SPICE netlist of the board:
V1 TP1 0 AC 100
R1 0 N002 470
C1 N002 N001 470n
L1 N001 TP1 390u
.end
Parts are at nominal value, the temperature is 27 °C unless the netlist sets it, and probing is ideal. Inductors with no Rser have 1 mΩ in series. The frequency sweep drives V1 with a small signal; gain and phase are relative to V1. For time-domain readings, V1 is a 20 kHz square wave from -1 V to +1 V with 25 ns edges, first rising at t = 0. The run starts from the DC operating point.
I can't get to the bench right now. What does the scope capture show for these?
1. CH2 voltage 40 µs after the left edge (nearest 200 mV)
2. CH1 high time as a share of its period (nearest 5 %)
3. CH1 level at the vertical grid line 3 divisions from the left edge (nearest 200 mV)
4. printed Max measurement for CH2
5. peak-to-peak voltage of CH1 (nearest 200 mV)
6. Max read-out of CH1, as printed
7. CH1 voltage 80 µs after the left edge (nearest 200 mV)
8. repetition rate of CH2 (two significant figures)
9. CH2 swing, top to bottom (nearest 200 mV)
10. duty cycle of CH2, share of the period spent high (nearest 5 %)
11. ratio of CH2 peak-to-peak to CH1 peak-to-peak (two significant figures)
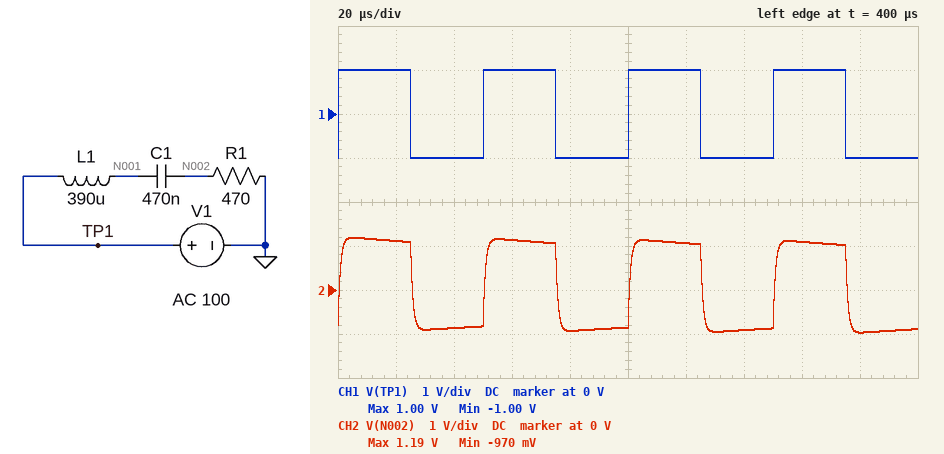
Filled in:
-800 mV
50 %
1.0 V
1.19 V
2.0 V
1.00 V
-1.0 V
20 kHz
2.2 V
50 %
1.1
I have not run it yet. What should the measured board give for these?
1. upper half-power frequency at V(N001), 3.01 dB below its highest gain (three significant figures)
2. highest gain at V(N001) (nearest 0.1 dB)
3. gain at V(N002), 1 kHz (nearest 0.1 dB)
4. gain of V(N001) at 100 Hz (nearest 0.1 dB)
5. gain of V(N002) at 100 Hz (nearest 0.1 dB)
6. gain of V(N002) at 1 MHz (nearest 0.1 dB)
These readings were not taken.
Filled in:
191 kHz
0 dB
-1.8 dB
0 dB
-17.2 dB
-14.5 dB
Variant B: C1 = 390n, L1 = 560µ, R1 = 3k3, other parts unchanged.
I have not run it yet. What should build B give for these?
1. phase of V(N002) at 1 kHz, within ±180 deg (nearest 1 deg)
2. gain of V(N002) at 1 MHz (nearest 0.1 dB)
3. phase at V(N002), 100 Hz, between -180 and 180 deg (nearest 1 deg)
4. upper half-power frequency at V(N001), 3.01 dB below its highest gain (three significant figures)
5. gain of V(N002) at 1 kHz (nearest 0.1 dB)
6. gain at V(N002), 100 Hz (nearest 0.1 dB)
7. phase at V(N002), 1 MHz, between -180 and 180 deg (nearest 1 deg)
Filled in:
7 deg
-3.3 dB
51 deg
938 kHz
-0.1 dB
-4.0 dB
-47 deg
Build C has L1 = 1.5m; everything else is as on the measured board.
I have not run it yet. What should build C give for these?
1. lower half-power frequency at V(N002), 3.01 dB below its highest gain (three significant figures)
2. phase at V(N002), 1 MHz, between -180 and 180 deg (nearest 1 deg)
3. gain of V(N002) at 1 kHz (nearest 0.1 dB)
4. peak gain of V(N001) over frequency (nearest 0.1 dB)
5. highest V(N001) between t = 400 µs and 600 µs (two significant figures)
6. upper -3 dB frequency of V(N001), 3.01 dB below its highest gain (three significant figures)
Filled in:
710 Hz
-87 deg
-1.7 dB
0.1 dB
1.0 V
49.4 kHz
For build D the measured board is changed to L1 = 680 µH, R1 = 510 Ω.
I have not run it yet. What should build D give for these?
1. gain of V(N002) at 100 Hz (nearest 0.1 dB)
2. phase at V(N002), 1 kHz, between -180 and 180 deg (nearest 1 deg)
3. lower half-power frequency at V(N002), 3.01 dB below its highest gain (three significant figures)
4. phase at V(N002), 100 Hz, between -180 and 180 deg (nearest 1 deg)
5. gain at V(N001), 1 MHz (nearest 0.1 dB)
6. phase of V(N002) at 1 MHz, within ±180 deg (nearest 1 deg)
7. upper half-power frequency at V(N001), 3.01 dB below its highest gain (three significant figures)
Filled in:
-16.5 dB
33 deg
660 Hz
81 deg
-18.5 dB
-83 deg
119 kHz
